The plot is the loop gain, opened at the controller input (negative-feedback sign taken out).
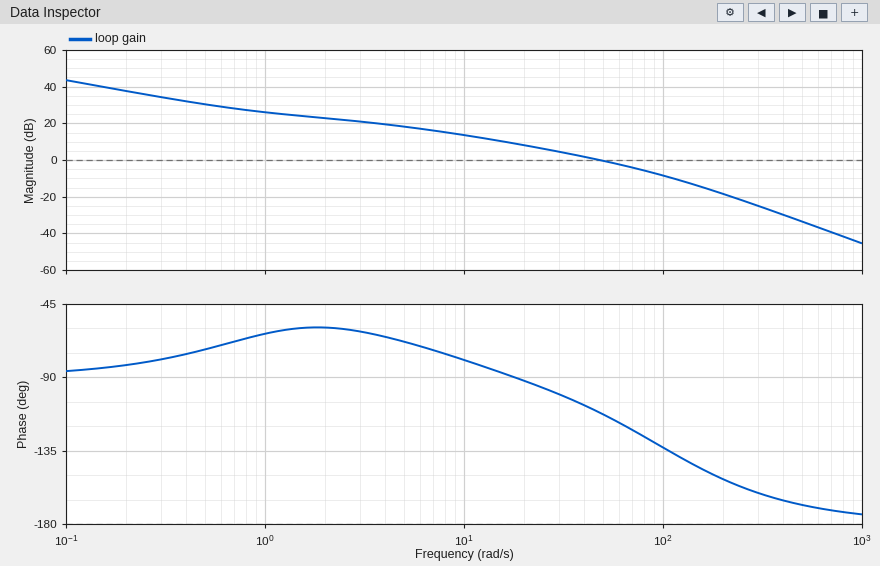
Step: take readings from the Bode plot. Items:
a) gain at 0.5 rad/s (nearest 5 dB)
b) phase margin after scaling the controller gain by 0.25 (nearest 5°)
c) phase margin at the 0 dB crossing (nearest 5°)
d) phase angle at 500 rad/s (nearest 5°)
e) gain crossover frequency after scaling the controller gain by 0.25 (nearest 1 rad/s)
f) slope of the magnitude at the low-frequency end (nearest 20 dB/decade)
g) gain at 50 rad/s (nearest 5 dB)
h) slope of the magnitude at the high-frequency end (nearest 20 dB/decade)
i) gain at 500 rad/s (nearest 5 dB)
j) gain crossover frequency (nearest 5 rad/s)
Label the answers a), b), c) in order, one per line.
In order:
a) 30 dB
b) 95°
c) 70°
d) -170°
e) 12 rad/s
f) -20 dB/decade
g) 0 dB
h) -40 dB/decade
i) -35 dB
j) 50 rad/s
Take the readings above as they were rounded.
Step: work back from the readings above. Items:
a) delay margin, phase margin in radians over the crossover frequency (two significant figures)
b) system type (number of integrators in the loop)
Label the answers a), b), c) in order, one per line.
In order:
a) 0.024 s
b) 1
